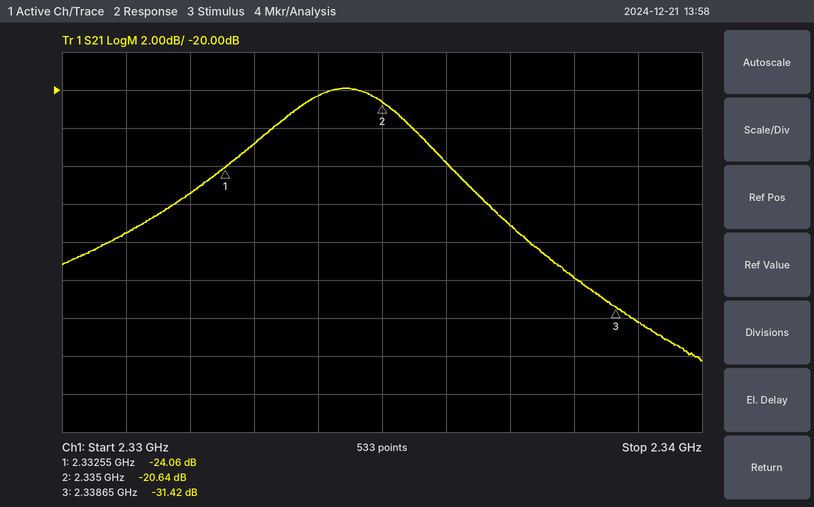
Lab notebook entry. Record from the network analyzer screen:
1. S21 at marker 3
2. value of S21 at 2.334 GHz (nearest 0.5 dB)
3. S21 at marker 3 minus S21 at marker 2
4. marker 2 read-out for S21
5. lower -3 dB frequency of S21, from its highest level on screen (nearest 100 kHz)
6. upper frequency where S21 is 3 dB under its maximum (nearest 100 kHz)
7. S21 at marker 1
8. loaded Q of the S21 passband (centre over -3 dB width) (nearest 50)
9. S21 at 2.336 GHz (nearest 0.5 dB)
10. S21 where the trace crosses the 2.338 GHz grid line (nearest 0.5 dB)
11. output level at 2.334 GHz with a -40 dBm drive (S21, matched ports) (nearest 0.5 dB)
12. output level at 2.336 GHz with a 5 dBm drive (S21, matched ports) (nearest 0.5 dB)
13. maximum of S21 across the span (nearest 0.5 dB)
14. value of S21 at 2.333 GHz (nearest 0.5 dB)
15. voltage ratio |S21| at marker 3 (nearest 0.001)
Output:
-31.42 dB
-20.5 dB
-10.78 dB
-20.64 dB
2.3330 GHz
2.3357 GHz
-24.06 dB
850
-24.0 dB
-30.0 dB
-60.5 dBm
-19.0 dBm
-20.0 dB
-23.0 dB
0.027
